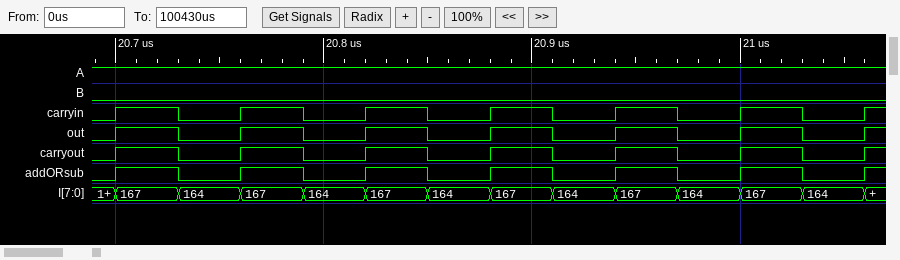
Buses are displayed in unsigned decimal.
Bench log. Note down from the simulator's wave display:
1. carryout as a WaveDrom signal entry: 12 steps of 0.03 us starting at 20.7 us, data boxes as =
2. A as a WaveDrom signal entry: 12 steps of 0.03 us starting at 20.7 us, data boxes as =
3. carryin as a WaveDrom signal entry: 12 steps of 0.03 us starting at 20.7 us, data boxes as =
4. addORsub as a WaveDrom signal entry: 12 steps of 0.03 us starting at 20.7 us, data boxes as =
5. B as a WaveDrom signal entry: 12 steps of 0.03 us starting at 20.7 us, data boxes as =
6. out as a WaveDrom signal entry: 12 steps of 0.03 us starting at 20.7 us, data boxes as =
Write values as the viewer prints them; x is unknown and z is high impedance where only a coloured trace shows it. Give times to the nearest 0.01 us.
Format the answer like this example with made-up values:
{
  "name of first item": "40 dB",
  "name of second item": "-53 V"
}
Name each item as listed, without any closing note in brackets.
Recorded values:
{
  "carryout as a WaveDrom signal entry: 12 steps of 0.03 us starting at 20.7 us, data boxes as =": "{name: 'carryout', wave: '101010101010'}",
  "A as a WaveDrom signal entry: 12 steps of 0.03 us starting at 20.7 us, data boxes as =": "{name: 'A', wave: '1...........'}",
  "carryin as a WaveDrom signal entry: 12 steps of 0.03 us starting at 20.7 us, data boxes as =": "{name: 'carryin', wave: '101010101010'}",
  "addORsub as a WaveDrom signal entry: 12 steps of 0.03 us starting at 20.7 us, data boxes as =": "{name: 'addORsub', wave: '101010101010'}",
  "B as a WaveDrom signal entry: 12 steps of 0.03 us starting at 20.7 us, data boxes as =": "{name: 'B', wave: '0...........'}",
  "out as a WaveDrom signal entry: 12 steps of 0.03 us starting at 20.7 us, data boxes as =": "{name: 'out', wave: '101010101010'}"
}
